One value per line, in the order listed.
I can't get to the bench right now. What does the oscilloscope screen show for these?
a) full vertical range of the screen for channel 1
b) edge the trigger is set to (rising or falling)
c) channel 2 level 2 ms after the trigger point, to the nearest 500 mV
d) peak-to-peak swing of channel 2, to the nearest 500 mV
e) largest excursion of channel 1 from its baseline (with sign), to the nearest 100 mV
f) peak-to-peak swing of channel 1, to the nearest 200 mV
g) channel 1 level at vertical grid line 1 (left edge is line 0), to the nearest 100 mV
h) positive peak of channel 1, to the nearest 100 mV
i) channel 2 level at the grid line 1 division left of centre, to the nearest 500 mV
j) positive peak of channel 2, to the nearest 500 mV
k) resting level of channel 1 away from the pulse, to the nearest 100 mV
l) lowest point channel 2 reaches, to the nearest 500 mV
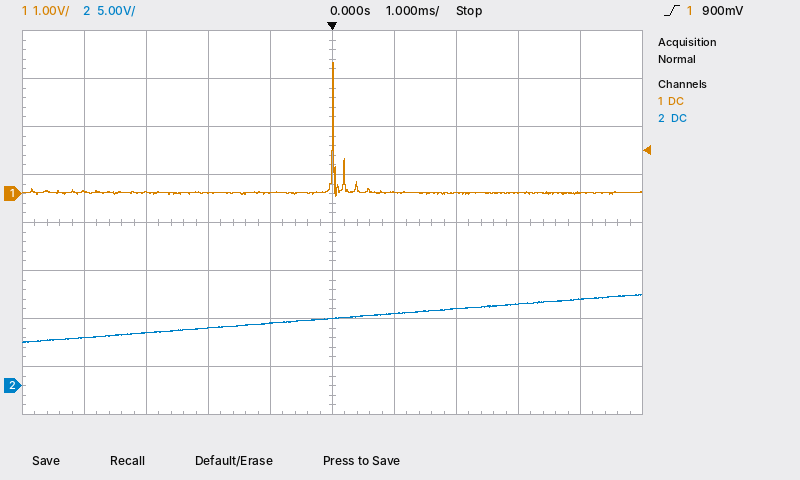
8 V
rising
8.0 V
5.0 V
+2.7 V
2.8 V
0.0 V
2.7 V
6.5 V
9.5 V
0.0 V
4.5 V
